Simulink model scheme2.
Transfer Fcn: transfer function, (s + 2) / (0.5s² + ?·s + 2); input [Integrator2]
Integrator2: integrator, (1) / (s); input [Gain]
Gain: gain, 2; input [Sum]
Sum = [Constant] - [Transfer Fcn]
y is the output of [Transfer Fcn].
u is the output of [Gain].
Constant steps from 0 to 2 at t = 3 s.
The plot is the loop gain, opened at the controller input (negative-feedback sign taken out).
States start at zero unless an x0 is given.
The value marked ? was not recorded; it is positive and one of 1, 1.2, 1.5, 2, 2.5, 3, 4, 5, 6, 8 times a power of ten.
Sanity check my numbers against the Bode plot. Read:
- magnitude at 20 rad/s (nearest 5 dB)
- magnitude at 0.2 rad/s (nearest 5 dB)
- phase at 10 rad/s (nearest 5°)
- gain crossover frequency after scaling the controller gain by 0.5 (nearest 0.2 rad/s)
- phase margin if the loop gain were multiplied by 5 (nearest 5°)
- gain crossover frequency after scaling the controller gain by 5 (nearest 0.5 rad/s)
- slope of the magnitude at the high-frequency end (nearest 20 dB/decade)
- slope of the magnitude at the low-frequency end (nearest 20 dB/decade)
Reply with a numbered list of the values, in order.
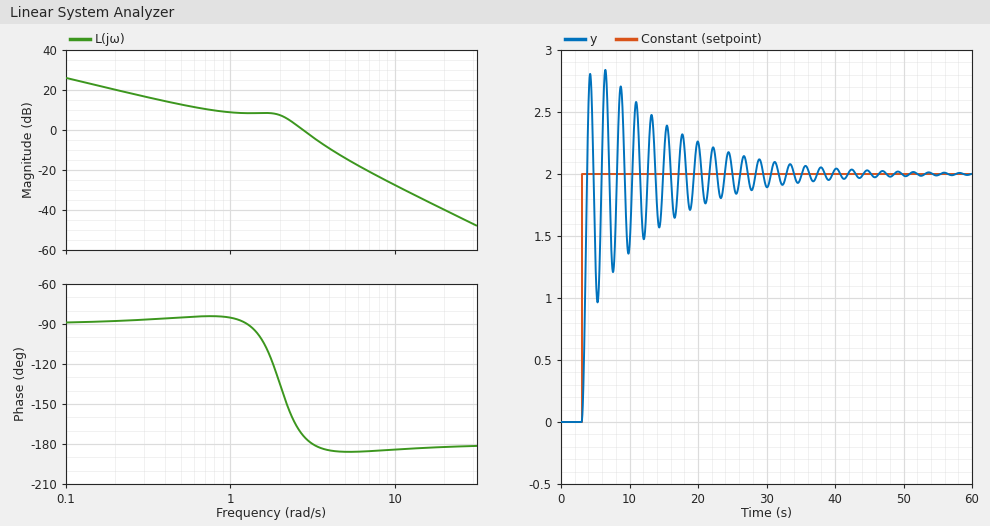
1. -40 dB
2. 20 dB
3. -185°
4. 2.2 rad/s
5. -5°
6. 5.0 rad/s
7. -40 dB/decade
8. -20 dB/decade
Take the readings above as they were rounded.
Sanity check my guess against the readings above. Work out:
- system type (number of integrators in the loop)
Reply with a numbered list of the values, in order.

1. 1
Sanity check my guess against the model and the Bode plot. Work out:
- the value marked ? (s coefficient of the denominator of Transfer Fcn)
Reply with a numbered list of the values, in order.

1. 0.6
